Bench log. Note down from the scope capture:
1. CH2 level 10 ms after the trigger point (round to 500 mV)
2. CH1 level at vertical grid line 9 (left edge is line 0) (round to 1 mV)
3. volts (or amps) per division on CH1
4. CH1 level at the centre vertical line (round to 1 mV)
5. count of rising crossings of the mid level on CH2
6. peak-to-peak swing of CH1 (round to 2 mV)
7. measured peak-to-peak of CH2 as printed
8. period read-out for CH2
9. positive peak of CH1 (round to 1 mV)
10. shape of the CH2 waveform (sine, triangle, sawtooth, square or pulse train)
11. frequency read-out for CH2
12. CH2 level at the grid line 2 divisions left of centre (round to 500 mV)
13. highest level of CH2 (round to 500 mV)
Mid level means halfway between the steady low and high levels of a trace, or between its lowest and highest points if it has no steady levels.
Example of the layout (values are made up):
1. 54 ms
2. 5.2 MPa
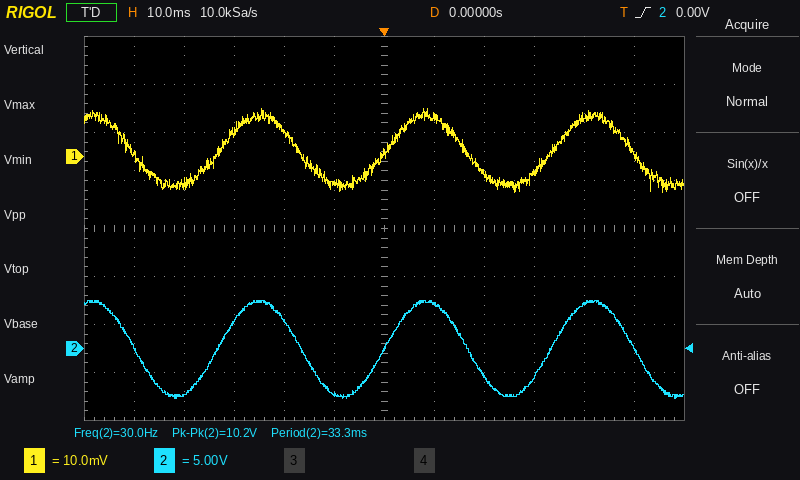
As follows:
1. 4.5 V
2. -3 mV
3. 10 mV
4. 1 mV
5. 3
6. 18 mV
7. 10.2 V
8. 33.3 ms
9. 10 mV
10. sine
11. 30.0 Hz
12. 3.0 V
13. 5.0 V
